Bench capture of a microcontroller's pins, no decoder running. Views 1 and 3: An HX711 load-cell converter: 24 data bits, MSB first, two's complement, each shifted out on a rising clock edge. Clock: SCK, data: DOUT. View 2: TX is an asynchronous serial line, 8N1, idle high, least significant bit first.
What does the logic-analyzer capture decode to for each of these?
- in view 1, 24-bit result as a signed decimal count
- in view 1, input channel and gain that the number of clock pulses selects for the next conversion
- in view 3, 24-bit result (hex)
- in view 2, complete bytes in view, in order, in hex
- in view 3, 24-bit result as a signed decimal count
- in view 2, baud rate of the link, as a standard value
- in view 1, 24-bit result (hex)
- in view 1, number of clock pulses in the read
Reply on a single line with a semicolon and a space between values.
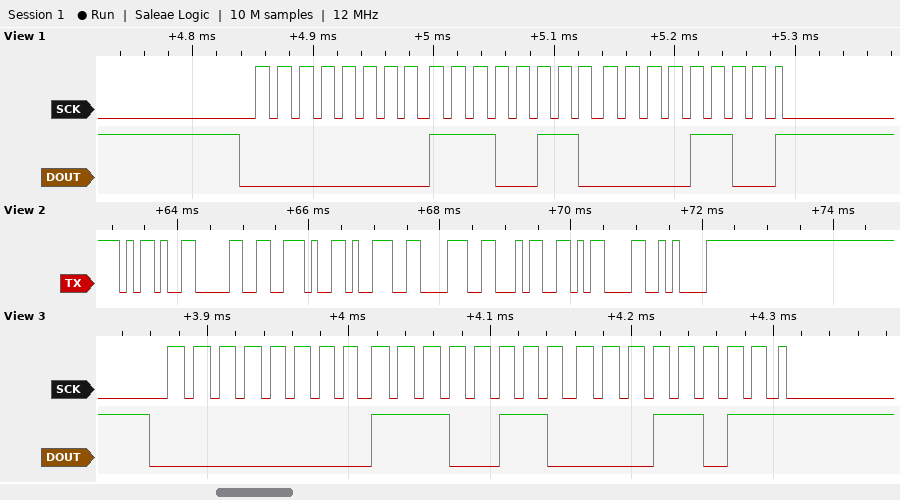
58892; channel A, gain 128; 0x00E61B; 2D 30 2E 39 38 34 0D 0A; 58907; 9600 baud; 0x00E60C; 25
